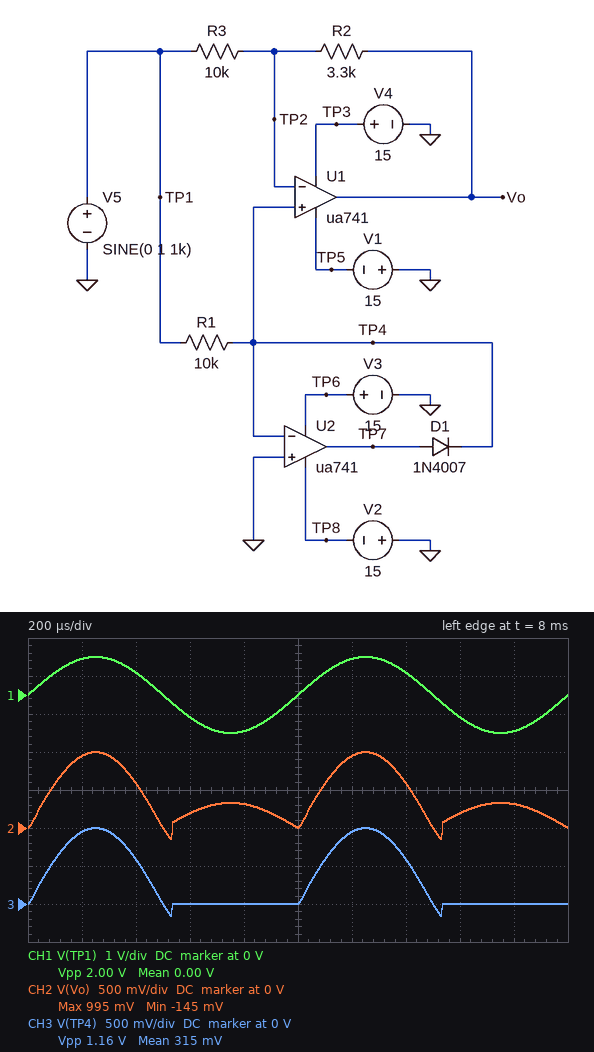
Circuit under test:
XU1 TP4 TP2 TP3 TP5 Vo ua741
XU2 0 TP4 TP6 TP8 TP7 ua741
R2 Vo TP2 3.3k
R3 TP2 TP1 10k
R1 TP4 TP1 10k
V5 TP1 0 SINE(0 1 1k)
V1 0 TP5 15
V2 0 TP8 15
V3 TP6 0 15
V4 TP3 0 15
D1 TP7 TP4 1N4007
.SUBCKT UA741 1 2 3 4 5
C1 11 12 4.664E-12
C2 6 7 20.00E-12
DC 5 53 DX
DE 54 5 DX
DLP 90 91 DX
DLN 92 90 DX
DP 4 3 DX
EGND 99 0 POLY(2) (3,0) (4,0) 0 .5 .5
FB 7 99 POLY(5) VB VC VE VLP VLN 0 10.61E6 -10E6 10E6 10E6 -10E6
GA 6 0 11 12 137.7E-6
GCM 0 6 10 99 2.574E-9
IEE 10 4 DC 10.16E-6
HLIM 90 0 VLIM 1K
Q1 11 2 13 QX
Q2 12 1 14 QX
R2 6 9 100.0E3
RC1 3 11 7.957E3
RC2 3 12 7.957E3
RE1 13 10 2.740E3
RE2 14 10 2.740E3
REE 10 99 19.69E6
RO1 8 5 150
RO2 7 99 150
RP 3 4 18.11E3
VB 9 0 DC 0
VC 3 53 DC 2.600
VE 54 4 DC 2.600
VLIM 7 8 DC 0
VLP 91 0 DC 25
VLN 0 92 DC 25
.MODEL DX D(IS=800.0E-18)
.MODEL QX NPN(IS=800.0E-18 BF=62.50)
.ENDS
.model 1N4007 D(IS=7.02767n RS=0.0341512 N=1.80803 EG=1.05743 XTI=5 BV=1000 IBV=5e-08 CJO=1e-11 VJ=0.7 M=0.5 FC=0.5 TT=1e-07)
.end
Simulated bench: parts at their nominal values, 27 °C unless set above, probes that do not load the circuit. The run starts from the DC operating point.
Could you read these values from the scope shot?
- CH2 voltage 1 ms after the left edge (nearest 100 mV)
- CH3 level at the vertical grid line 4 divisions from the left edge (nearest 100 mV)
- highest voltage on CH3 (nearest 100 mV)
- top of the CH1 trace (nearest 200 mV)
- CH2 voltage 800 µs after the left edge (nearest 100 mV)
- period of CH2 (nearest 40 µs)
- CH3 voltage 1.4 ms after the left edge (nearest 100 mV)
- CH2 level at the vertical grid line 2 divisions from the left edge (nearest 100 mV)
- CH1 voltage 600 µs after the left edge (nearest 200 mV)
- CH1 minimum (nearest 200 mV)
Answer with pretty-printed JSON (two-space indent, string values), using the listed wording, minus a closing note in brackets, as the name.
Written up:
{
  "CH2 voltage 1 ms after the left edge": "0 V",
  "CH3 level at the vertical grid line 4 divisions from the left edge": "0 V",
  "highest voltage on CH3": "1.0 V",
  "top of the CH1 trace": "1.0 V",
  "CH2 voltage 800 µs after the left edge": "300 mV",
  "period of CH2": "1.00 ms",
  "CH3 voltage 1.4 ms after the left edge": "600 mV",
  "CH2 level at the vertical grid line 2 divisions from the left edge": "600 mV",
  "CH1 voltage 600 µs after the left edge": "-600 mV",
  "CH1 minimum": "-1.0 V"
}
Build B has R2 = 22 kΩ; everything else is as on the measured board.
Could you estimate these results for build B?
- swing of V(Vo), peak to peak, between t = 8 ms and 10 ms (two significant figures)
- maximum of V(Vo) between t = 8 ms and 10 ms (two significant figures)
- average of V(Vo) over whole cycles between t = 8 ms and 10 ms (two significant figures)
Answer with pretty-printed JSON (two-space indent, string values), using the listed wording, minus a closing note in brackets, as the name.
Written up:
{
  "swing of V(Vo), peak to peak, between t = 8 ms and 10 ms": "2.3 V",
  "maximum of V(Vo) between t = 8 ms and 10 ms": "2.2 V",
  "average of V(Vo) over whole cycles between t = 8 ms and 10 ms": "1.0 V"
}
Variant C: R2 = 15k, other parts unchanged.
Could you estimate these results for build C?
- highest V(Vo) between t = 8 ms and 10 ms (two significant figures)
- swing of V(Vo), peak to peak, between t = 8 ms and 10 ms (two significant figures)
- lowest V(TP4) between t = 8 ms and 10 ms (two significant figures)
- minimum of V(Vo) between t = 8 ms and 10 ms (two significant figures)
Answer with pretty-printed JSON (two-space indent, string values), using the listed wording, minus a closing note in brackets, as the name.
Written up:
{
  "highest V(Vo) between t = 8 ms and 10 ms": "1.5 V",
  "swing of V(Vo), peak to peak, between t = 8 ms and 10 ms": "1.6 V",
  "lowest V(TP4) between t = 8 ms and 10 ms": "-160 mV",
  "minimum of V(Vo) between t = 8 ms and 10 ms": "-110 mV"
}
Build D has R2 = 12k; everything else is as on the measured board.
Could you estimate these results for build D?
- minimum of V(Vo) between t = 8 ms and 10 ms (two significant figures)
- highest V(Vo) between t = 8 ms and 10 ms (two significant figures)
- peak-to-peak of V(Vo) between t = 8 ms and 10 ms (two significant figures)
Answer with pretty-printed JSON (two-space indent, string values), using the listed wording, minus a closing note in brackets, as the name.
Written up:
{
  "minimum of V(Vo) between t = 8 ms and 10 ms": "-120 mV",
  "highest V(Vo) between t = 8 ms and 10 ms": "1.2 V",
  "peak-to-peak of V(Vo) between t = 8 ms and 10 ms": "1.3 V"
}
